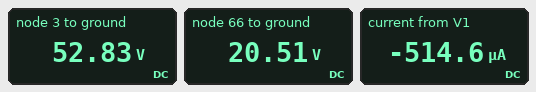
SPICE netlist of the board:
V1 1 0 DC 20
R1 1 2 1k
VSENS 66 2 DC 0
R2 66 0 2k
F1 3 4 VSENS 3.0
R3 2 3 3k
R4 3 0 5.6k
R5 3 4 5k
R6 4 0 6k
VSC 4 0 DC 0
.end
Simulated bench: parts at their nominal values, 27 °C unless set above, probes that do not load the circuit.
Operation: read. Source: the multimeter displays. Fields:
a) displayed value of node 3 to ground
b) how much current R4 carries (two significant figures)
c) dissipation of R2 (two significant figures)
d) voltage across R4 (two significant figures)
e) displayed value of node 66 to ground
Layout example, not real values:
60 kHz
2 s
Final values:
52.83 V
9.4 mA
210 mW
53 V
20.51 V
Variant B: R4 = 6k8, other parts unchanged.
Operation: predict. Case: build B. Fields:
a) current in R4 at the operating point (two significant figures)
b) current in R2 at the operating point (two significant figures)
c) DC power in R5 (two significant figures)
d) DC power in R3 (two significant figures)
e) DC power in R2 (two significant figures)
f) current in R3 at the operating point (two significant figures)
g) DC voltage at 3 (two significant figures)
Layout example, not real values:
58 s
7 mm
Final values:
8.5 mA
11 mA
660 mW
440 mW
230 mW
12 mA
58 V
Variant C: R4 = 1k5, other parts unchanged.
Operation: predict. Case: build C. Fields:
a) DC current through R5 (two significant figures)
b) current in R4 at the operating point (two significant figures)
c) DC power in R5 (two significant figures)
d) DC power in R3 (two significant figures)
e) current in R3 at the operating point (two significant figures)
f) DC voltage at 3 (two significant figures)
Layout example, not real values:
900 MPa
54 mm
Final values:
4.6 mA
15 mA
110 mW
21 mW
2.7 mA
23 V
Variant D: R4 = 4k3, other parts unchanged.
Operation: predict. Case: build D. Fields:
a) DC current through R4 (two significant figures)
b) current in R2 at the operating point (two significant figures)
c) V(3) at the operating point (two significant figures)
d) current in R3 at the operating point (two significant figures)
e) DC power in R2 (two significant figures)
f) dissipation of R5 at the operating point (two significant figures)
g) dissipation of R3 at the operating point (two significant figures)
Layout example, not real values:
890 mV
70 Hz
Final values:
11 mA
9.7 mA
46 V
9.0 mA
190 mW
430 mW
240 mW
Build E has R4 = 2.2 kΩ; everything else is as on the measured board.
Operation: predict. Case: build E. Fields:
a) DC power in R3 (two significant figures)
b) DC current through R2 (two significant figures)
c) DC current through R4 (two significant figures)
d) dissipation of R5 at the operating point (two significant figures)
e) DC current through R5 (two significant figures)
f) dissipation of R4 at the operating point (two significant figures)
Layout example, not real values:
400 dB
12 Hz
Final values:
66 mW
8.2 mA
14 mA
190 mW
6.1 mA
420 mW
